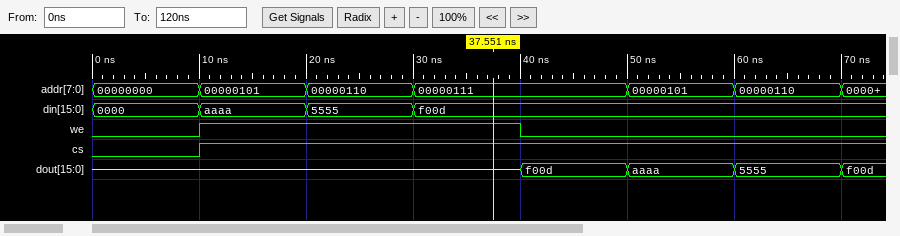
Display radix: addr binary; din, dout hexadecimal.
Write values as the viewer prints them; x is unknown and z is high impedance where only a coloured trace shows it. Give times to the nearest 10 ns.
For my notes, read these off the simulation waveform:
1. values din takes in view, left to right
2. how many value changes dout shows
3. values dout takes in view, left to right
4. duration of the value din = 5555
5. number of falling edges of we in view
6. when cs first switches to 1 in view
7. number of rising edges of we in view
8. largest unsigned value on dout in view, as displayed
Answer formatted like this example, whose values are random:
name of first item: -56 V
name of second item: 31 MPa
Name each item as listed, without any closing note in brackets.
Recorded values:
values din takes in view, left to right: 0000, aaaa, 5555, f00d
how many value changes dout shows: 4
values dout takes in view, left to right: z, f00d, aaaa, 5555, f00d
duration of the value din = 5555: 10 ns
number of falling edges of we in view: 1
when cs first switches to 1 in view: 10 ns
number of rising edges of we in view: 1
largest unsigned value on dout in view, as displayed: f00d
